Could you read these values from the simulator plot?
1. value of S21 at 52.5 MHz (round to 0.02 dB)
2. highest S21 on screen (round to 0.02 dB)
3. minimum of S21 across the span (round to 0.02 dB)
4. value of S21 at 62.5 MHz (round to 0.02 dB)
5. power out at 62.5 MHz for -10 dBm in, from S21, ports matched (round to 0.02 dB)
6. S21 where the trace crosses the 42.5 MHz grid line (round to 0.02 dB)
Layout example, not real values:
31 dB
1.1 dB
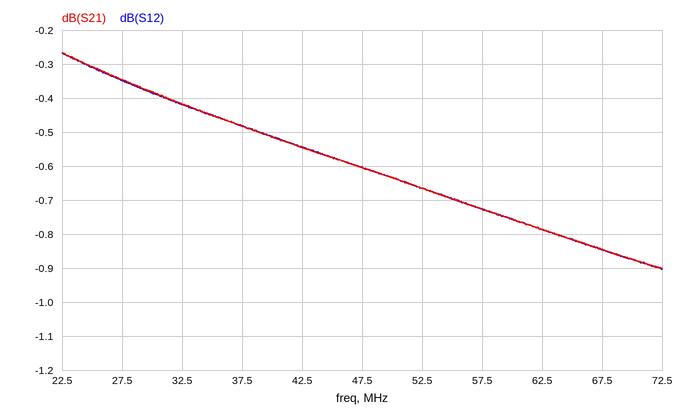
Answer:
-0.66 dB
-0.26 dB
-0.90 dB
-0.78 dB
-10.78 dBm
-0.54 dB
